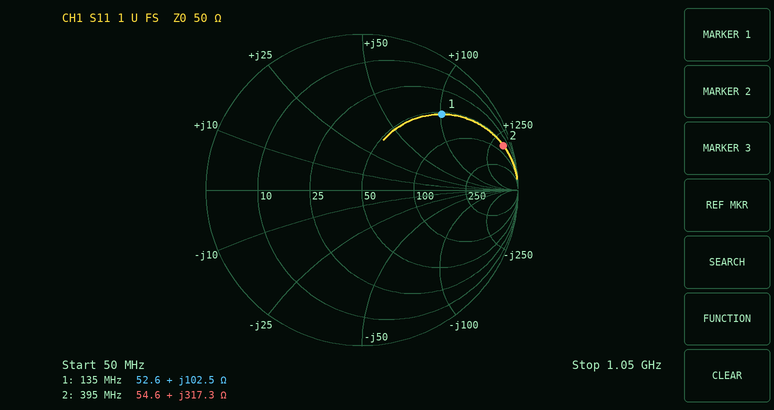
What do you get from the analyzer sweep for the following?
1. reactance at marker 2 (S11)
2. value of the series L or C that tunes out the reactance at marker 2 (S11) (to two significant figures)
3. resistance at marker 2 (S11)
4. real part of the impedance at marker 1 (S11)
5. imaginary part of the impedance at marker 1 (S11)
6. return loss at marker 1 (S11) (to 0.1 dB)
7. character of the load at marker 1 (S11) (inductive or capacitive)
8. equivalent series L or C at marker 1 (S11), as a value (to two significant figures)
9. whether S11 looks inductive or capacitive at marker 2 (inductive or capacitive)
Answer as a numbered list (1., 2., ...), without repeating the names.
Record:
1. +317.3 Ω
2. 1.3 pF
3. 54.6 Ω
4. 52.6 Ω
5. +102.5 Ω
6. 3.0 dB
7. inductive
8. 120 nH
9. inductive
